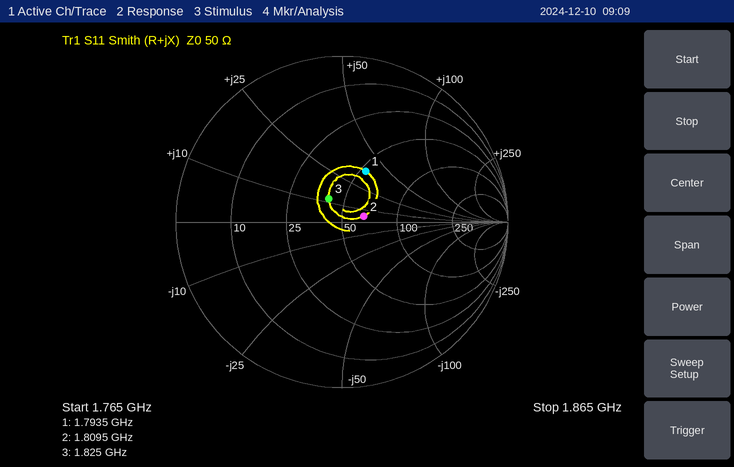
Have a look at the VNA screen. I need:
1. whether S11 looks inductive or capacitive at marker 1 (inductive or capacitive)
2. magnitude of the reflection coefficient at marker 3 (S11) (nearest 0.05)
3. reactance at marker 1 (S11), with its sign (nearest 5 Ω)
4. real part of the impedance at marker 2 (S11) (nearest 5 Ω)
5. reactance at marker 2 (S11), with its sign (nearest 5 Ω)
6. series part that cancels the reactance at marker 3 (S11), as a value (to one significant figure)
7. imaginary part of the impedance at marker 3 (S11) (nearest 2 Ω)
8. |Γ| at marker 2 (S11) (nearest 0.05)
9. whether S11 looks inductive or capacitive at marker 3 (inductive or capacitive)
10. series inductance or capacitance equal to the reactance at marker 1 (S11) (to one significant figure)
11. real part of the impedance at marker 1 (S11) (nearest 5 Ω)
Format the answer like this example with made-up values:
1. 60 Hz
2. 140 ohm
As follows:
1. inductive
2. 0.15
3. +35 Ω
4. 65 Ω
5. +5 Ω
6. 7 pF
7. +12 Ω
8. 0.15
9. inductive
10. 3 nH
11. 55 Ω
